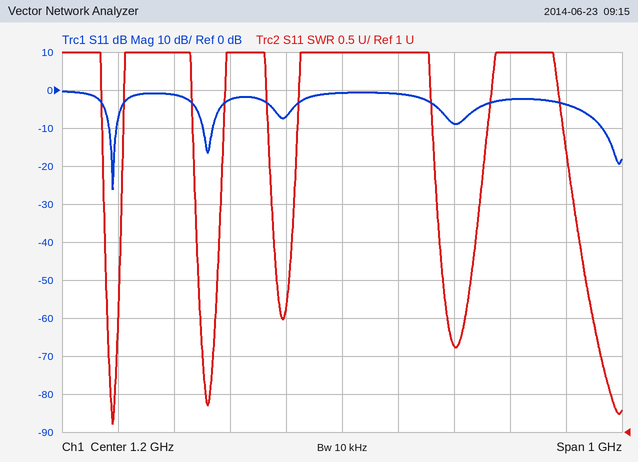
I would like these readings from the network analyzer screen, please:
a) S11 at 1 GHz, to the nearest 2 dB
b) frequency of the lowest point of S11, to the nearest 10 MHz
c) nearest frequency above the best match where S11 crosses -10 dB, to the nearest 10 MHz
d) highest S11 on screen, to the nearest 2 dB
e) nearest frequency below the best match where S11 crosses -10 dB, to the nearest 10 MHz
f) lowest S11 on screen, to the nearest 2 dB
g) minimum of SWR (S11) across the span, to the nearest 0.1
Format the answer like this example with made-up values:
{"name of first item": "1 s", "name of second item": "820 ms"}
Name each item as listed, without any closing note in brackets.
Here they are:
{"S11 at 1 GHz, to the nearest 2 dB": "-2 dB", "frequency of the lowest point of S11, to the nearest 10 MHz": "790 MHz", "nearest frequency above the best match where S11 crosses -10 dB, to the nearest 10 MHz": "800 MHz", "highest S11 on screen, to the nearest 2 dB": "0 dB", "nearest frequency below the best match where S11 crosses -10 dB, to the nearest 10 MHz": "780 MHz", "lowest S11 on screen, to the nearest 2 dB": "-26 dB", "minimum of SWR (S11) across the span, to the nearest 0.1": "1.1"}
